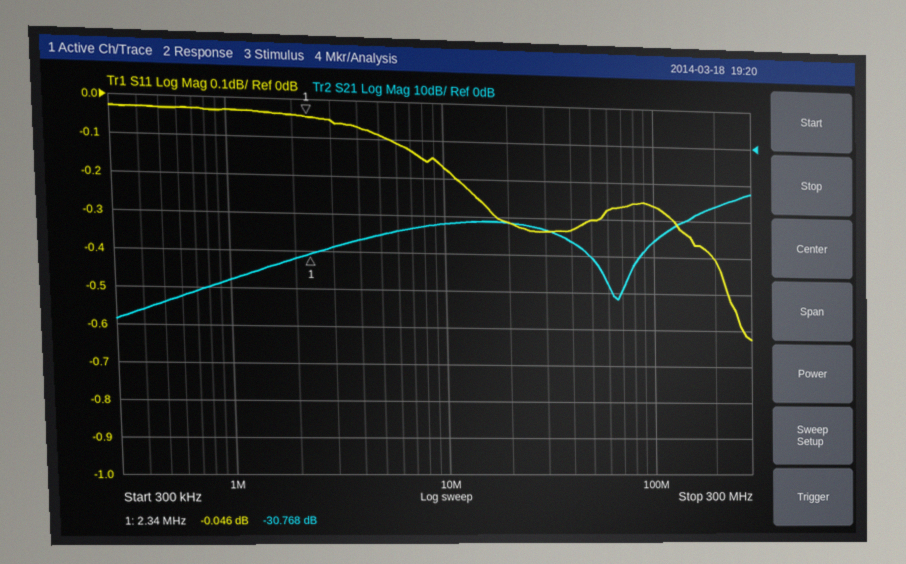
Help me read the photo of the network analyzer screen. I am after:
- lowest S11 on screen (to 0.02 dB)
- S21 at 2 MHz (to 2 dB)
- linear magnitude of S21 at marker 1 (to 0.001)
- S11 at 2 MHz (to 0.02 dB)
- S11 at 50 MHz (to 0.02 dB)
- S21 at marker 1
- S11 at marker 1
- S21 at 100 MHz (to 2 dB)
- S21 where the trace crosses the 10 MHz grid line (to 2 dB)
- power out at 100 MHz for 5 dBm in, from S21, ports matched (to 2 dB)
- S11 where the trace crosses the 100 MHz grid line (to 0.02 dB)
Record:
-0.62 dB
-32 dB
0.029
-0.04 dB
-0.30 dB
-30.768 dB
-0.046 dB
-26 dB
-22 dB
-20 dBm
-0.26 dB
